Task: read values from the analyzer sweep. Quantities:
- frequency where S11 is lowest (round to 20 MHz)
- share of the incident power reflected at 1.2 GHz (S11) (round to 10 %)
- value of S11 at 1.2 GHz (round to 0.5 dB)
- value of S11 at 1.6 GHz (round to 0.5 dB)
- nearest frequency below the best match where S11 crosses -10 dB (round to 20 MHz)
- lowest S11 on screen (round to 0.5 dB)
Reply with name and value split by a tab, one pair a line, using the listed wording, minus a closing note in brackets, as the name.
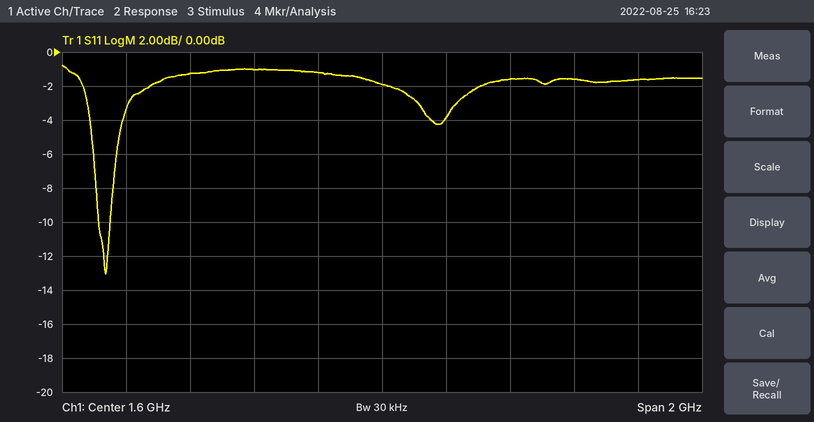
frequency where S11 is lowest	740 MHz
share of the incident power reflected at 1.2 GHz (S11)	80 %
value of S11 at 1.2 GHz	-1.0 dB
value of S11 at 1.6 GHz	-2.0 dB
nearest frequency below the best match where S11 crosses -10 dB	720 MHz
lowest S11 on screen	-13.0 dB
